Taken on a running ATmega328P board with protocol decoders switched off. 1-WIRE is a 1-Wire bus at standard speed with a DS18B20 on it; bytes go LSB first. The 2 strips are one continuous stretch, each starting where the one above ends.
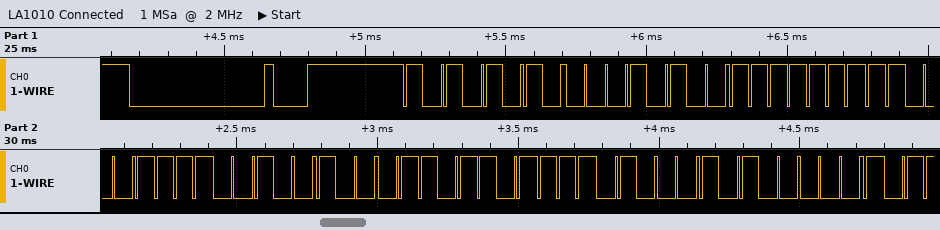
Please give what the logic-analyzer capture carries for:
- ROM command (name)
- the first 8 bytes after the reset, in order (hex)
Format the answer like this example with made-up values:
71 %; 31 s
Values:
Match ROM; 55 28 FF F1 24 B6 17 05
